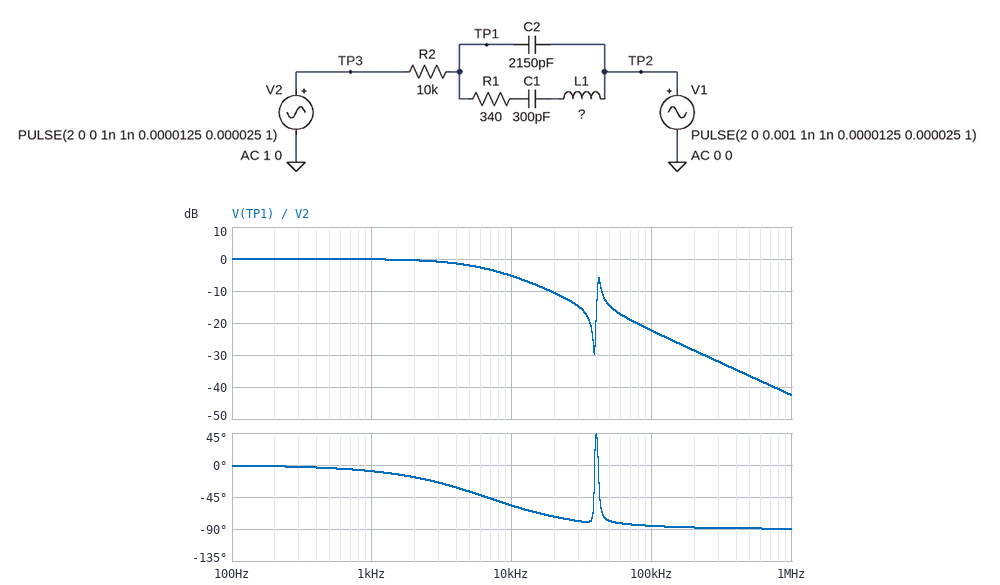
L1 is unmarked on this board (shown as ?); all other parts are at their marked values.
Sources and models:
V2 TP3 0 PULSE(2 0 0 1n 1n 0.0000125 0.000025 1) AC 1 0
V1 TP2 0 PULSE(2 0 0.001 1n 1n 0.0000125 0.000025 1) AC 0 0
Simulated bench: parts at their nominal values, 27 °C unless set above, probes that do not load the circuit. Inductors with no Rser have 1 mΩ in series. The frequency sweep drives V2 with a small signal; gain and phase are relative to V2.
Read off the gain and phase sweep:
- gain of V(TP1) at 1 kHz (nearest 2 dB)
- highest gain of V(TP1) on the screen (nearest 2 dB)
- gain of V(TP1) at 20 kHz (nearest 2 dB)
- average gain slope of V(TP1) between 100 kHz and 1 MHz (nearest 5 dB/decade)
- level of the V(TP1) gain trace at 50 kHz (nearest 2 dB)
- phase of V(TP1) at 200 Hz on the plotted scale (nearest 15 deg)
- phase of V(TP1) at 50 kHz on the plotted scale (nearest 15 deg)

0 dB
0 dB
-10 dB
-20 dB/decade
-14 dB
0 deg
-75 deg
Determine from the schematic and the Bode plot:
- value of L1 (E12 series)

56 mH
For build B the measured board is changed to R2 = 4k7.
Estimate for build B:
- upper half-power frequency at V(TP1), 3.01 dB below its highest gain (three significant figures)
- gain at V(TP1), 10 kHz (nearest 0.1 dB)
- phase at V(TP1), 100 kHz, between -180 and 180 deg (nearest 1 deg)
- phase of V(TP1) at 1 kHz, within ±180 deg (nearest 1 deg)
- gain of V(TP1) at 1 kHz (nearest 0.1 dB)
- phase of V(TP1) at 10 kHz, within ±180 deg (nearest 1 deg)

13.6 kHz
-1.9 dB
-81 deg
-4 deg
0 dB
-36 deg
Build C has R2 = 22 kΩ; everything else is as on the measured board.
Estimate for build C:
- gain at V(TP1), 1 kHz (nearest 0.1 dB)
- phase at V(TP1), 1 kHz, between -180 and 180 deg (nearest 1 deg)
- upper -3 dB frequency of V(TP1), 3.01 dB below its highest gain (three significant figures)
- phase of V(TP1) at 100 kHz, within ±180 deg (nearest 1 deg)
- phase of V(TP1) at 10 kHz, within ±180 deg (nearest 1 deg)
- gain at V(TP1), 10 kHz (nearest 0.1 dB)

-0.5 dB
-19 deg
2.95 kHz
-88 deg
-74 deg
-11.0 dB
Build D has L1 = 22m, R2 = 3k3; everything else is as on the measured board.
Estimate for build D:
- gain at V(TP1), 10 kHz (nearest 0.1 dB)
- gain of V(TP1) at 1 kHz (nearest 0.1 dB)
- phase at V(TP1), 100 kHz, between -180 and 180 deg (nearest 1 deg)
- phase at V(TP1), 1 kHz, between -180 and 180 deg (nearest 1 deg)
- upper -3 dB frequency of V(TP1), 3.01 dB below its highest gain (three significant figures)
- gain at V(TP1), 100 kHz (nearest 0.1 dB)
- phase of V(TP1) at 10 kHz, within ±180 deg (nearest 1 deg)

-1.0 dB
0 dB
-76 deg
-3 deg
19.4 kHz
-12.5 dB
-27 deg
